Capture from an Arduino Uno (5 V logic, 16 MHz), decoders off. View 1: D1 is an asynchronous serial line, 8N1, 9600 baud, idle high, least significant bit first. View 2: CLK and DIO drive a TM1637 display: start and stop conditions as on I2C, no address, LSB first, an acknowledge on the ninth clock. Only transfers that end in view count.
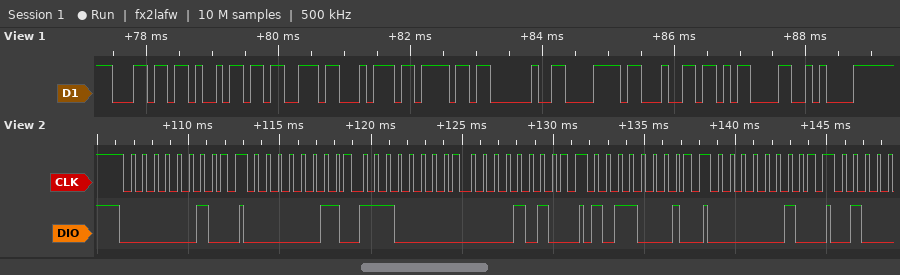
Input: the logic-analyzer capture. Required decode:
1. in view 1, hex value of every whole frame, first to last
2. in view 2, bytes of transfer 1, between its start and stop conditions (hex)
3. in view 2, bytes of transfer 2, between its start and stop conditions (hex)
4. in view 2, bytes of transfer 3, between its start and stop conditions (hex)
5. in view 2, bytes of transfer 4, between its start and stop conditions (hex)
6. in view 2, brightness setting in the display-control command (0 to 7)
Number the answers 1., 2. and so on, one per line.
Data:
1. 6C 69 73 74 6F 20 78 64 0D 0A
2. 40
3. C0 07 50
4. 8D
5. 40
6. 5
